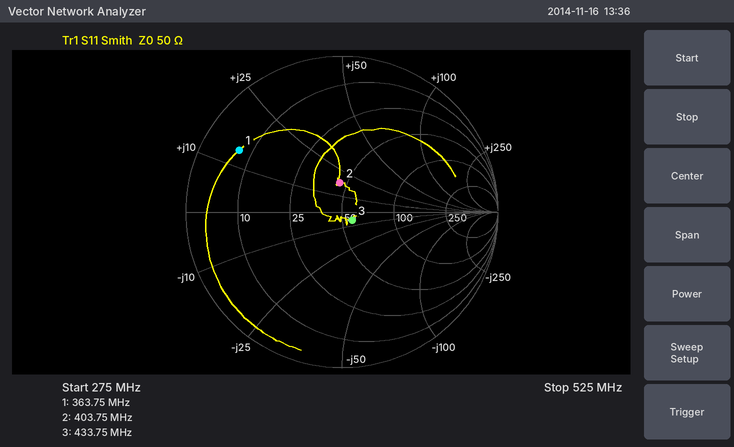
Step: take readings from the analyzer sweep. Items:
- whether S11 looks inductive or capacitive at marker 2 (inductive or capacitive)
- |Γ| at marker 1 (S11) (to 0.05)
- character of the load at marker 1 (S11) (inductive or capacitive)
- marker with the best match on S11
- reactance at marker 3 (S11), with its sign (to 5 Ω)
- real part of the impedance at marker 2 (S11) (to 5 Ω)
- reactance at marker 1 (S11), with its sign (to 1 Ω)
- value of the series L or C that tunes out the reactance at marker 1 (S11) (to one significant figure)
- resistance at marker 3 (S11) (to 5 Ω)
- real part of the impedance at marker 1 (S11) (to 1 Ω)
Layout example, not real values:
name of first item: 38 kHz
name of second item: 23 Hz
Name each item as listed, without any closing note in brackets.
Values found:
whether S11 looks inductive or capacitive at marker 2: inductive
|Γ| at marker 1 (S11): 0.75
character of the load at marker 1 (S11): inductive
marker with the best match on S11: marker 3
reactance at marker 3 (S11), with its sign: -5 Ω
real part of the impedance at marker 2 (S11): 45 Ω
reactance at marker 1 (S11), with its sign: +14 Ω
value of the series L or C that tunes out the reactance at marker 1 (S11): 30 pF
resistance at marker 3 (S11): 55 Ω
real part of the impedance at marker 1 (S11): 7 Ω
